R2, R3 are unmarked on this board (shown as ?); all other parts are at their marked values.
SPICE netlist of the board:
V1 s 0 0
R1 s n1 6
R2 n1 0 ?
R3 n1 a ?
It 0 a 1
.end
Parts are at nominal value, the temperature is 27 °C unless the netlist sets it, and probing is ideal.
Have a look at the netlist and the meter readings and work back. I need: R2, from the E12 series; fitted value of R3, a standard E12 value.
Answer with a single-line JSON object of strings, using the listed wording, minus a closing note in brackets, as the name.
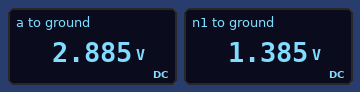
{"R2, from the E12 series": "1.8 Ω", "fitted value of R3, a standard E12 value": "1.5 Ω"}
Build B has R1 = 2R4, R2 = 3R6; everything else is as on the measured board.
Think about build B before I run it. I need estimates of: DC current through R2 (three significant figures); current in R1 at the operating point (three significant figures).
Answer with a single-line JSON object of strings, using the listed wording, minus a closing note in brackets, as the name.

{"DC current through R2": "400 mA", "current in R1 at the operating point": "600 mA"}
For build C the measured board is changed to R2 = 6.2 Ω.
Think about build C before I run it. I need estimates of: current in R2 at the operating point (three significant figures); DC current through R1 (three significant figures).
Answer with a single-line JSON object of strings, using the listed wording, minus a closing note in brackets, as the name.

{"current in R2 at the operating point": "492 mA", "DC current through R1": "508 mA"}
